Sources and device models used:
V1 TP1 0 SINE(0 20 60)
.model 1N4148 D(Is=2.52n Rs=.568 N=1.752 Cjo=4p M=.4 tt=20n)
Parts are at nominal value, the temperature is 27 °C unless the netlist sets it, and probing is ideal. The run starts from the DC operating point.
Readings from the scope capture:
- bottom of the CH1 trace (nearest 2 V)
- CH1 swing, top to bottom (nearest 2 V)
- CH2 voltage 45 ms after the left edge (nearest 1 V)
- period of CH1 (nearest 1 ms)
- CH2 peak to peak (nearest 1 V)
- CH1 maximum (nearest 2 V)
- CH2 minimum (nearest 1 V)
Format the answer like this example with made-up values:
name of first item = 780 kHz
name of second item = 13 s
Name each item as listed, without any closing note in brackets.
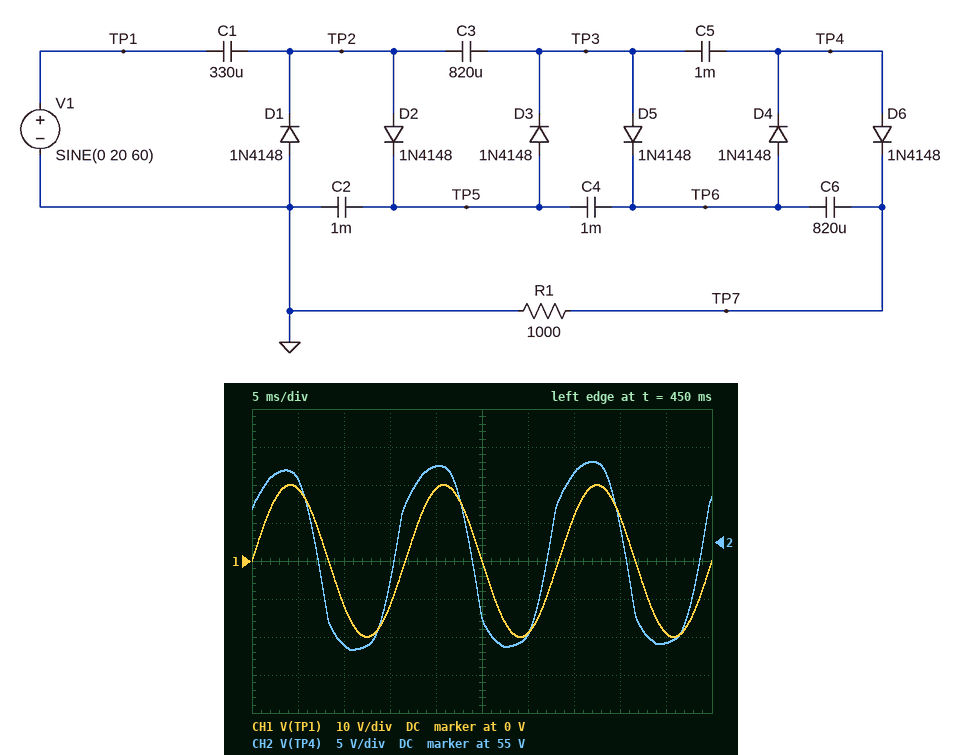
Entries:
bottom of the CH1 trace = -20 V
CH1 swing, top to bottom = 40 V
CH2 voltage 45 ms after the left edge = 42 V
period of CH1 = 17 ms
CH2 peak to peak = 25 V
CH1 maximum = 20 V
CH2 minimum = 41 V
